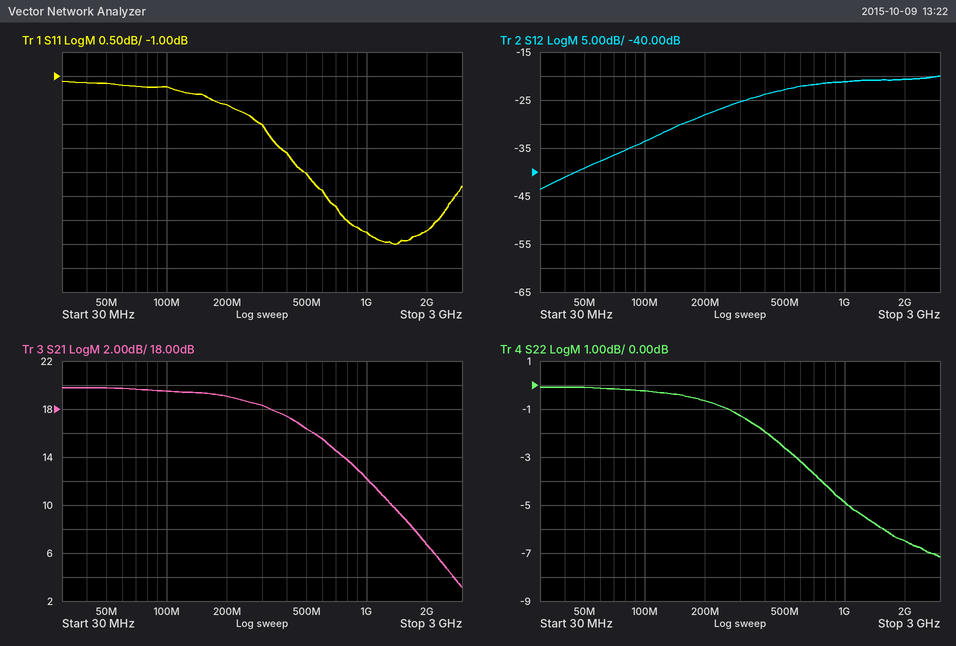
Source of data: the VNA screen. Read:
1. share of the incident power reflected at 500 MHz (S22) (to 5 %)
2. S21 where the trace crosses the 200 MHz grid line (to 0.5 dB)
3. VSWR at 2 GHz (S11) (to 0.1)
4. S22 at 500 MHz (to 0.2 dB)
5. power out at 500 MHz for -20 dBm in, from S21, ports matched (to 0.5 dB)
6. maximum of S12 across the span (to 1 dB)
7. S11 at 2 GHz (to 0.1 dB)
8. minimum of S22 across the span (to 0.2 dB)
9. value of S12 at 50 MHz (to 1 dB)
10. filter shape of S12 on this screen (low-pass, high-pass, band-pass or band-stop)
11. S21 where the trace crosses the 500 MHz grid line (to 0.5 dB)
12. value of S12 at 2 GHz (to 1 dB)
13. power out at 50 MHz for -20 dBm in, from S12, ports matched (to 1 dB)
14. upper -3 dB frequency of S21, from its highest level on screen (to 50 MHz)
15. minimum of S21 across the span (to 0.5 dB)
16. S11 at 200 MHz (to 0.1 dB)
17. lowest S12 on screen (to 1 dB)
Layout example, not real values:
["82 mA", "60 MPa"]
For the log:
["55 %", "19.0 dB", "4.2", "-2.6 dB", "-3.5 dBm", "-20 dB", "-4.2 dB", "-7.2 dB", "-39 dB", "high-pass", "16.5 dB", "-21 dB", "-59 dBm", "450 MHz", "3.0 dB", "-1.6 dB", "-44 dB"]
